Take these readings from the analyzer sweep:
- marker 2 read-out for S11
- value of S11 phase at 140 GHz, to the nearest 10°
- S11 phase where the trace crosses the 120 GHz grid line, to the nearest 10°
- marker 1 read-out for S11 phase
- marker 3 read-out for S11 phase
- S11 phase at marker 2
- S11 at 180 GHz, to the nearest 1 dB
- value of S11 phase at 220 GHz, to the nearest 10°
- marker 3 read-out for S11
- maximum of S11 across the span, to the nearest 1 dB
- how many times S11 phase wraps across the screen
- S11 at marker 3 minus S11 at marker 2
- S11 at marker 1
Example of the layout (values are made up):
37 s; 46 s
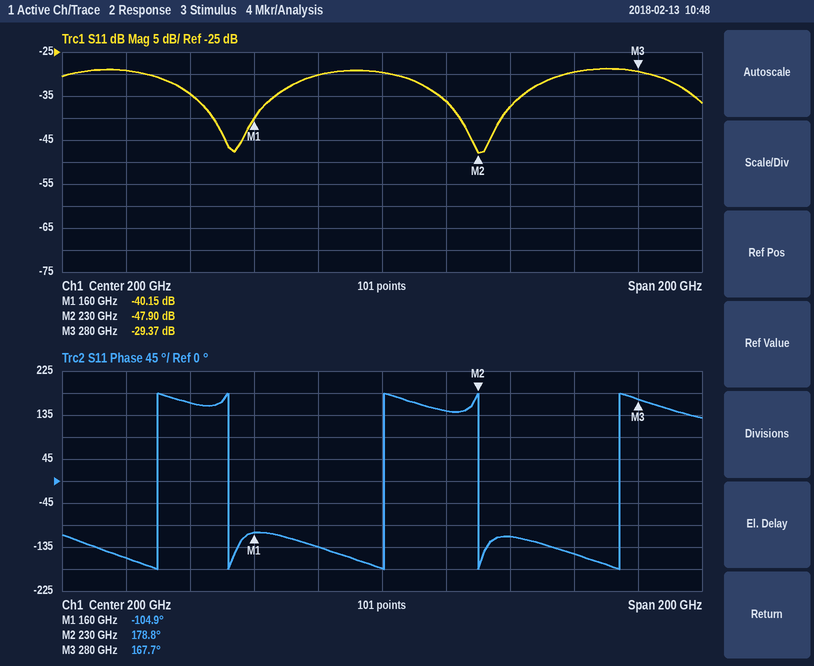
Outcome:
-47.90 dB; 160°; -160°; -104.9°; 167.7°; 178.8°; -30 dB; 140°; -29.37 dB; -29 dB; 5; 18.53 dB; -40.15 dB
